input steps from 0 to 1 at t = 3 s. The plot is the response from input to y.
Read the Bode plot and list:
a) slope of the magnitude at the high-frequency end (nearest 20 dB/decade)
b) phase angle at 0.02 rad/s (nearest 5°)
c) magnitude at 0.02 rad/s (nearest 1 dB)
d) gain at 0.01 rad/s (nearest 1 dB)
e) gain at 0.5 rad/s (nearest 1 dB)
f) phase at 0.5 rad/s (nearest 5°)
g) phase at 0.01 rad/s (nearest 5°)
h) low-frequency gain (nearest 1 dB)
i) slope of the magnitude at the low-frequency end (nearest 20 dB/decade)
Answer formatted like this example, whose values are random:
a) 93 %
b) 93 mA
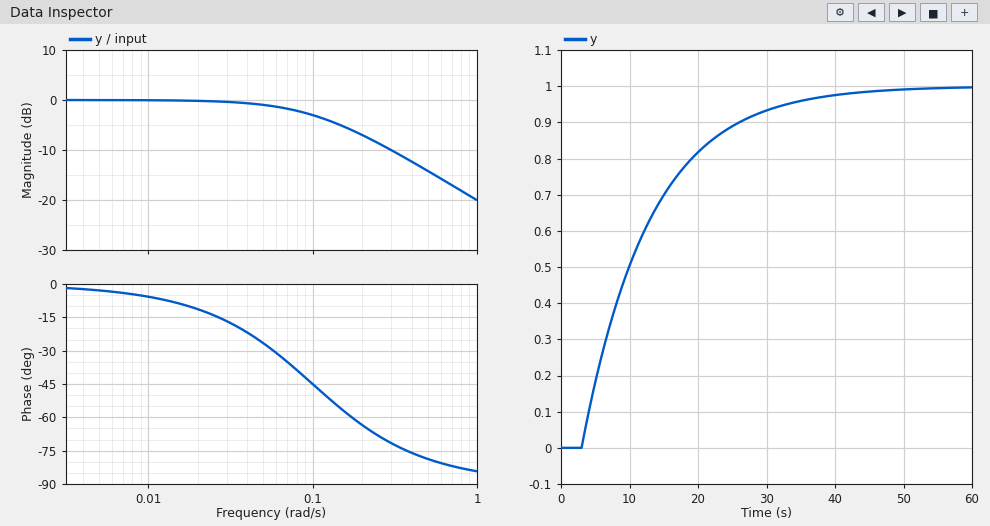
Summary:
a) -20 dB/decade
b) -10°
c) 0 dB
d) 0 dB
e) -14 dB
f) -80°
g) -5°
h) 0 dB
i) 0 dB/decade
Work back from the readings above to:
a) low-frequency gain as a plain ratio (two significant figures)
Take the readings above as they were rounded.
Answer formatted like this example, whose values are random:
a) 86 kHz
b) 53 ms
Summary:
a) 1.0
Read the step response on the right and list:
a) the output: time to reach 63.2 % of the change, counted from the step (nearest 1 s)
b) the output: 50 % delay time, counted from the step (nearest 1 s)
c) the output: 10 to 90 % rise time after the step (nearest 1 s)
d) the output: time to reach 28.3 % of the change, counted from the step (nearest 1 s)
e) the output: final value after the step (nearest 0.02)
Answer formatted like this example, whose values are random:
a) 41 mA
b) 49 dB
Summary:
a) 10 s
b) 7 s
c) 22 s
d) 3 s
e) 1.00
